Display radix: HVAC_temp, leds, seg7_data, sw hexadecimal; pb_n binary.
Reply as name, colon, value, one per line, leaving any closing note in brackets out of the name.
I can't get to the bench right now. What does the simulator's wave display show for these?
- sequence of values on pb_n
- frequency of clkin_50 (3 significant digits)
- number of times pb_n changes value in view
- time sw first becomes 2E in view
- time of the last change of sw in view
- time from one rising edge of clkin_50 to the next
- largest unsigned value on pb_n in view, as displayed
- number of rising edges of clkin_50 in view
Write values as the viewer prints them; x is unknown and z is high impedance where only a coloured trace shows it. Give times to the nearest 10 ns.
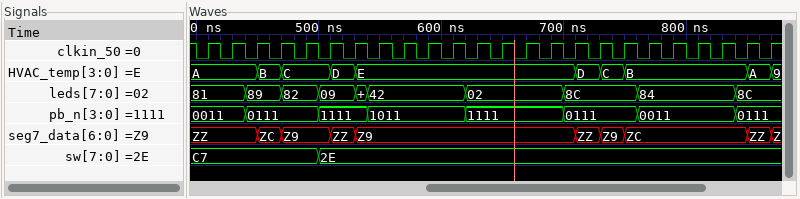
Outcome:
sequence of values on pb_n: 0011, 0111, 1111, 1011, 1111, 0111, 0011, 0111
frequency of clkin_50: 50.0 MHz
number of times pb_n changes value in view: 7
time sw first becomes 2E in view: 500 ns
time of the last change of sw in view: 500 ns
time from one rising edge of clkin_50 to the next: 20 ns
largest unsigned value on pb_n in view, as displayed: 1111
number of rising edges of clkin_50 in view: 24
